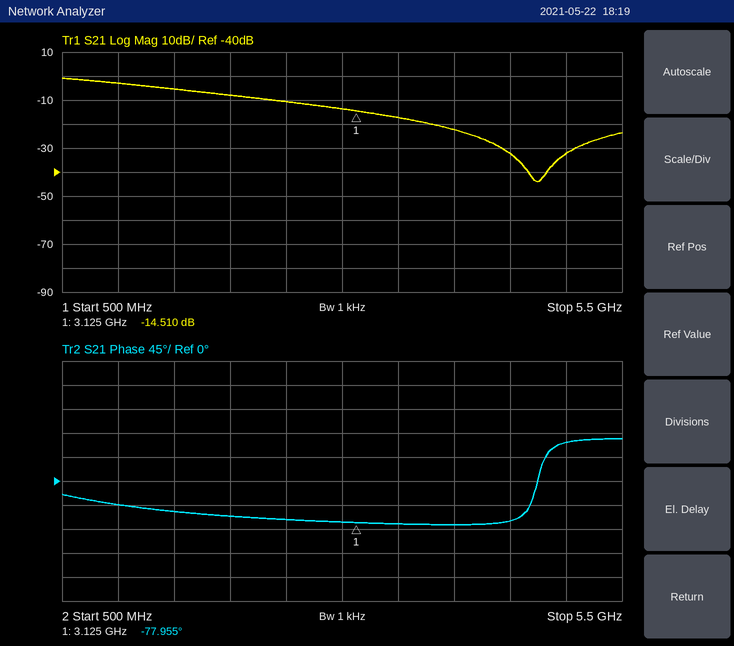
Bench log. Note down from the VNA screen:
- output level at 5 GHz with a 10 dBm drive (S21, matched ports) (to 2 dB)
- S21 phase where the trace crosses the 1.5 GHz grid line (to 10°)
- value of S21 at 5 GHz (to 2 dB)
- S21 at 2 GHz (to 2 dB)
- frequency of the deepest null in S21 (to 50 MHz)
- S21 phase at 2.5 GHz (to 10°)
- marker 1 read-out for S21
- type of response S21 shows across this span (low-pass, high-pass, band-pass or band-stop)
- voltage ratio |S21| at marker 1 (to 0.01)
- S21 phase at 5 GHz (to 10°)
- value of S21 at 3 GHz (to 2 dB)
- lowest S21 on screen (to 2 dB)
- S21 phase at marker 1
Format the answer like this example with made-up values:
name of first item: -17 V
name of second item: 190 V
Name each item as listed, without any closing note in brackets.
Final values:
output level at 5 GHz with a 10 dBm drive (S21, matched ports): -22 dBm
S21 phase where the trace crosses the 1.5 GHz grid line: -60°
value of S21 at 5 GHz: -32 dB
S21 at 2 GHz: -8 dB
frequency of the deepest null in S21: 4.75 GHz
S21 phase at 2.5 GHz: -70°
marker 1 read-out for S21: -14.510 dB
type of response S21 shows across this span: low-pass
voltage ratio |S21| at marker 1: 0.19
S21 phase at 5 GHz: 70°
value of S21 at 3 GHz: -14 dB
lowest S21 on screen: -44 dB
S21 phase at marker 1: -77.955°
